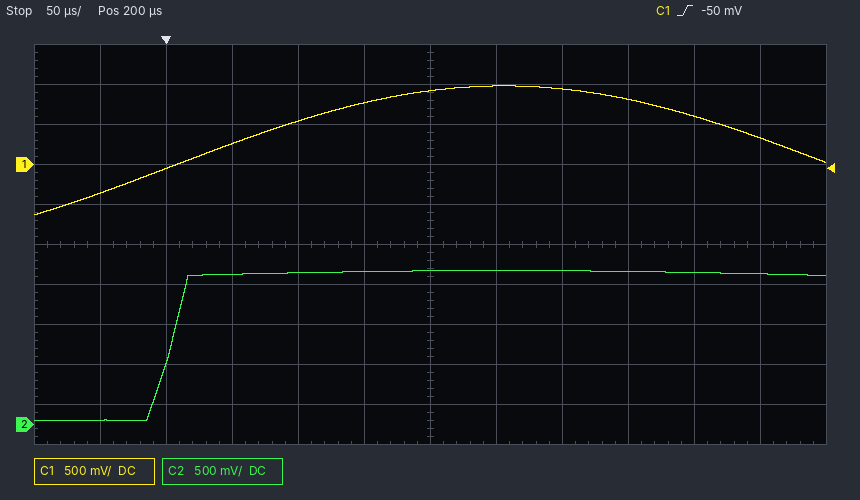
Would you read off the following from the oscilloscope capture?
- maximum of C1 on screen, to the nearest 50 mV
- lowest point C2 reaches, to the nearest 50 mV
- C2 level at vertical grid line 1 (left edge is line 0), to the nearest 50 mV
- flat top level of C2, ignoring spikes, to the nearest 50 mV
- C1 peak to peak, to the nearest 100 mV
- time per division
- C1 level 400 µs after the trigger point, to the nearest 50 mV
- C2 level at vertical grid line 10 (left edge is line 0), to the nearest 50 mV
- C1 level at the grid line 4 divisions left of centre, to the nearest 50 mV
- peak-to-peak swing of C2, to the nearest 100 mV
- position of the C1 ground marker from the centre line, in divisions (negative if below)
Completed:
1.00 V
50 mV
50 mV
1.90 V
1.60 V
50 µs
600 mV
1.90 V
-50 mV
1.90 V
+2.0 div
